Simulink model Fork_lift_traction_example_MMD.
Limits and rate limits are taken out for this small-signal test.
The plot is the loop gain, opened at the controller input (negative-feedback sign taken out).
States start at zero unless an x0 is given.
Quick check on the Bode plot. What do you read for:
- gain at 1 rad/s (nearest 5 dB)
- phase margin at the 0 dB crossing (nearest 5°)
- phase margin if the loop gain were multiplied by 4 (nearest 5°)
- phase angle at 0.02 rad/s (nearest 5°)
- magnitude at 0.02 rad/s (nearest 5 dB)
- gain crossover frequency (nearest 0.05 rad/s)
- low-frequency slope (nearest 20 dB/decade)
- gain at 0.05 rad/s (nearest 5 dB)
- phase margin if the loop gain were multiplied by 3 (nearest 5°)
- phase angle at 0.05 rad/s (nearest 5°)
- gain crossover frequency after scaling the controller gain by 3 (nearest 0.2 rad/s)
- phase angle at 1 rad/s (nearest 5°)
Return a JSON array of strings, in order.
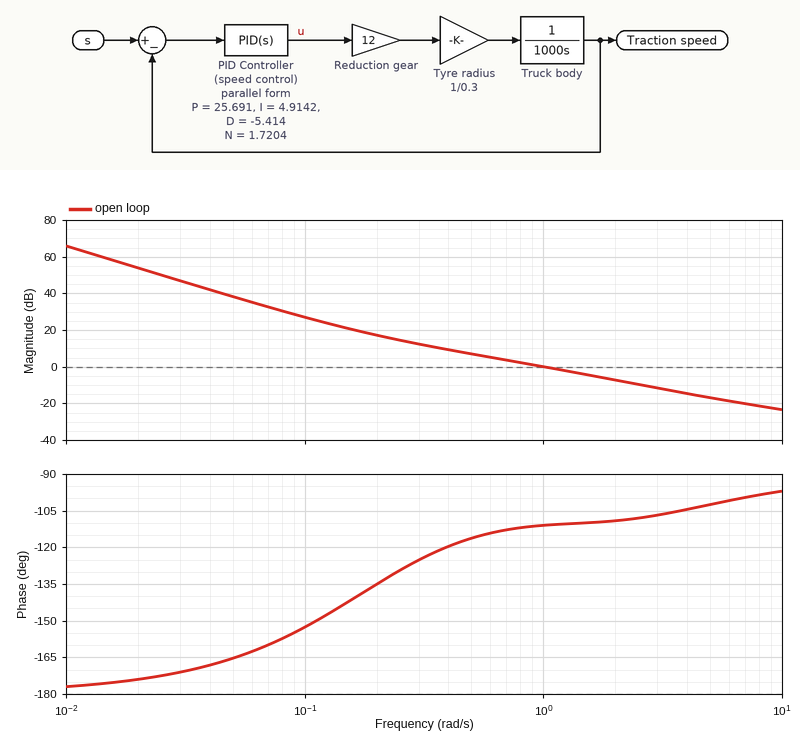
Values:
["0 dB", "70°", "75°", "-175°", "55 dB", "1.00 rad/s", "-40 dB/decade", "40 dB", "70°", "-165°", "2.4 rad/s", "-110°"]
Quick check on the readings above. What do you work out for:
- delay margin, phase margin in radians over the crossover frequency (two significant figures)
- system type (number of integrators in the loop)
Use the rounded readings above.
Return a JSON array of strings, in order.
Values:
["1.2 s", "2"]
